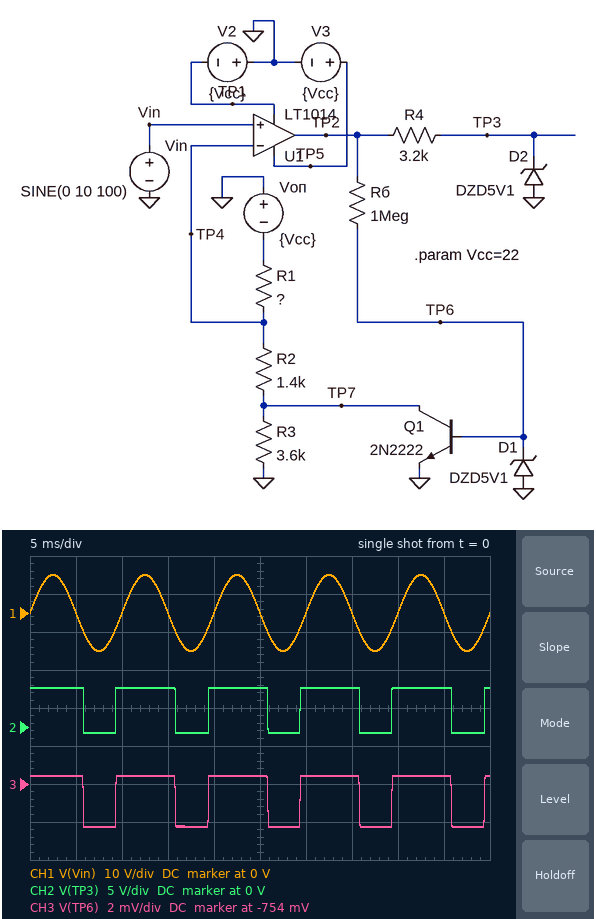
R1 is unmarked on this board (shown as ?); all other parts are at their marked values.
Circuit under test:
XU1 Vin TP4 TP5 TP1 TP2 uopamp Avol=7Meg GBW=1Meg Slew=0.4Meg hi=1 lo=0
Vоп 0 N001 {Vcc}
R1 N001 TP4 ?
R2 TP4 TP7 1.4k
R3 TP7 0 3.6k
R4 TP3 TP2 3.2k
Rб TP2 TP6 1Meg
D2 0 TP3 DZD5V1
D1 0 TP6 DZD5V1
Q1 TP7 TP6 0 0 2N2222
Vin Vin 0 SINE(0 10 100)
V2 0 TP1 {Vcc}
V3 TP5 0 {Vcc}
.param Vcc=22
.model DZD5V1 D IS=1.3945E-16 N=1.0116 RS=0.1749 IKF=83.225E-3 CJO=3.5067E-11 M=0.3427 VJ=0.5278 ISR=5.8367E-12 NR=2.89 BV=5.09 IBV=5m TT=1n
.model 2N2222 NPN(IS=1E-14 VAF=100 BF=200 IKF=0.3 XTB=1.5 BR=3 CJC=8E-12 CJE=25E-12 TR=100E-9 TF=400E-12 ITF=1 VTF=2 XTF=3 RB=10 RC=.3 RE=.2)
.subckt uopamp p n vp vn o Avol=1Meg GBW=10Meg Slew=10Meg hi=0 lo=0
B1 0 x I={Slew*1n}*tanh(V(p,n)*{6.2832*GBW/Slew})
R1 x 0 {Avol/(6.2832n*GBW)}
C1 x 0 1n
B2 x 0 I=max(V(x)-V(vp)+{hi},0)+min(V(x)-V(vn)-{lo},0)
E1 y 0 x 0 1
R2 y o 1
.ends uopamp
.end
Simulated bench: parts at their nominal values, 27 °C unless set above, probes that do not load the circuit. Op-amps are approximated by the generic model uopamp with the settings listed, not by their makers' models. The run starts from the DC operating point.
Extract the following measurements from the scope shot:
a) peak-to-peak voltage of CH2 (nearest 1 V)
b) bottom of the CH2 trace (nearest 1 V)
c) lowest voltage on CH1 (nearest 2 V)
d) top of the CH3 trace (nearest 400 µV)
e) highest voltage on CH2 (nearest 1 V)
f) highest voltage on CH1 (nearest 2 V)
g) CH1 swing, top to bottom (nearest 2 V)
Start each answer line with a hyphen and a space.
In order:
- 6 V
- -1 V
- -10 V
- -753.6 mV
- 5 V
- 10 V
- 20 V
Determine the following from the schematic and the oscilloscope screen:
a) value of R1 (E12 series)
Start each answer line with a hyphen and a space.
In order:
- 8.2 kΩ
